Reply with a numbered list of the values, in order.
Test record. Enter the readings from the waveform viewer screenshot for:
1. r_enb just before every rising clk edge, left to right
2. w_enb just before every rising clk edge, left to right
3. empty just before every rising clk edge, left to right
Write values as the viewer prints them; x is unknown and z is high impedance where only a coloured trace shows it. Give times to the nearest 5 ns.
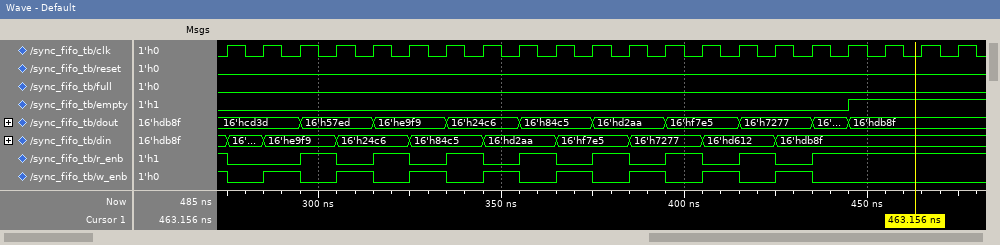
1. 1 0 0 1 0 1 0 1 0 1 0 1 0 1 0 1 0 1 1 1 1
2. 1 0 1 0 1 0 1 0 1 0 1 0 1 0 1 0 1 0 0 0 0
3. 0 0 0 0 0 0 0 0 0 0 0 0 0 0 0 0 0 0 1 1 1
